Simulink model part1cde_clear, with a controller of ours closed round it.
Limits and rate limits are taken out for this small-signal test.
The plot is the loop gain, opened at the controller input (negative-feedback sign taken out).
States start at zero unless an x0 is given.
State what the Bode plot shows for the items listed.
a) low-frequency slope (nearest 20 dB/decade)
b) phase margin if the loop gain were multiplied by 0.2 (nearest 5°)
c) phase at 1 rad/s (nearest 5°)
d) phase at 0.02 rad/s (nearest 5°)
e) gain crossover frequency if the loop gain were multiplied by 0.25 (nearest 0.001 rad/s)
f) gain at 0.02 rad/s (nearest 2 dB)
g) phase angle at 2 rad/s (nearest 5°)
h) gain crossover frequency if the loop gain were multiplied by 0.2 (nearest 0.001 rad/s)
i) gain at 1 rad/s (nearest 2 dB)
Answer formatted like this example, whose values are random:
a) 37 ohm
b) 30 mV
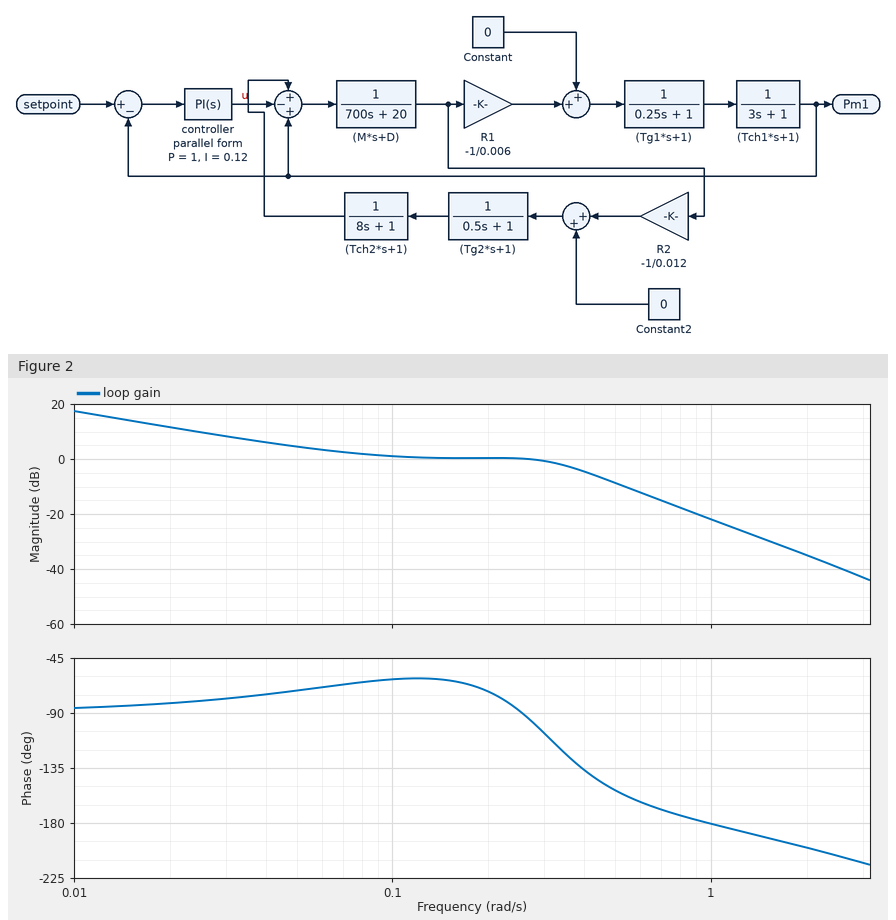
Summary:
a) -20 dB/decade
b) 95°
c) -180°
d) -80°
e) 0.019 rad/s
f) 12 dB
g) -200°
h) 0.015 rad/s
i) -22 dB
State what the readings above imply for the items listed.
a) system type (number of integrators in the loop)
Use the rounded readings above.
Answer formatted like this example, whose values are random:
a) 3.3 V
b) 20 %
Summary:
a) 1
